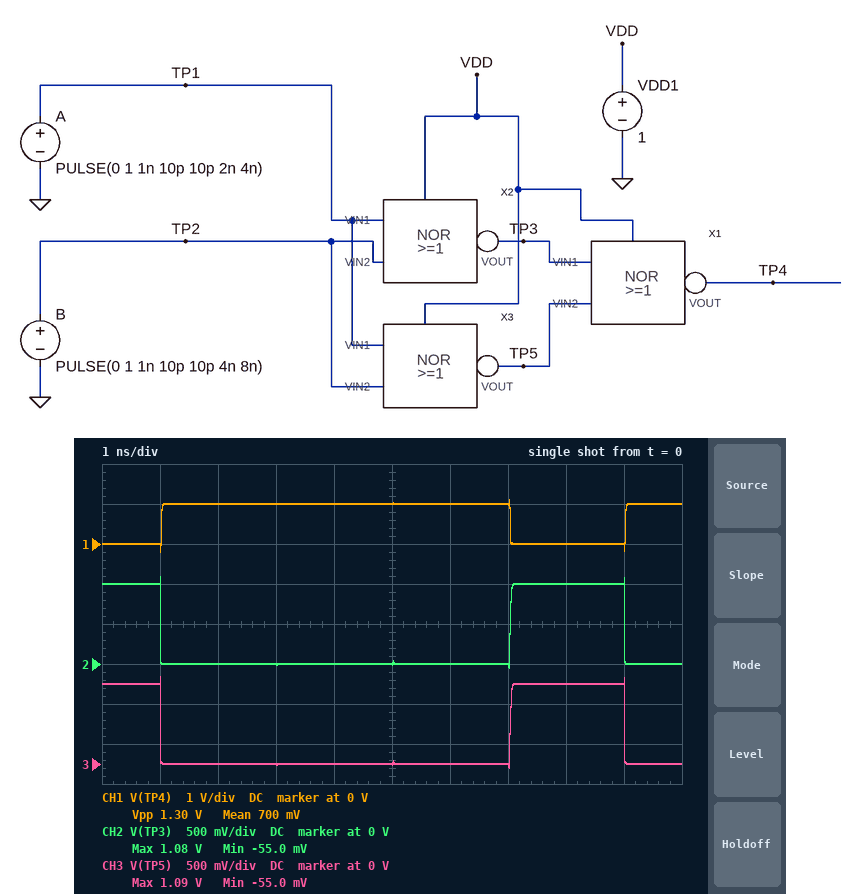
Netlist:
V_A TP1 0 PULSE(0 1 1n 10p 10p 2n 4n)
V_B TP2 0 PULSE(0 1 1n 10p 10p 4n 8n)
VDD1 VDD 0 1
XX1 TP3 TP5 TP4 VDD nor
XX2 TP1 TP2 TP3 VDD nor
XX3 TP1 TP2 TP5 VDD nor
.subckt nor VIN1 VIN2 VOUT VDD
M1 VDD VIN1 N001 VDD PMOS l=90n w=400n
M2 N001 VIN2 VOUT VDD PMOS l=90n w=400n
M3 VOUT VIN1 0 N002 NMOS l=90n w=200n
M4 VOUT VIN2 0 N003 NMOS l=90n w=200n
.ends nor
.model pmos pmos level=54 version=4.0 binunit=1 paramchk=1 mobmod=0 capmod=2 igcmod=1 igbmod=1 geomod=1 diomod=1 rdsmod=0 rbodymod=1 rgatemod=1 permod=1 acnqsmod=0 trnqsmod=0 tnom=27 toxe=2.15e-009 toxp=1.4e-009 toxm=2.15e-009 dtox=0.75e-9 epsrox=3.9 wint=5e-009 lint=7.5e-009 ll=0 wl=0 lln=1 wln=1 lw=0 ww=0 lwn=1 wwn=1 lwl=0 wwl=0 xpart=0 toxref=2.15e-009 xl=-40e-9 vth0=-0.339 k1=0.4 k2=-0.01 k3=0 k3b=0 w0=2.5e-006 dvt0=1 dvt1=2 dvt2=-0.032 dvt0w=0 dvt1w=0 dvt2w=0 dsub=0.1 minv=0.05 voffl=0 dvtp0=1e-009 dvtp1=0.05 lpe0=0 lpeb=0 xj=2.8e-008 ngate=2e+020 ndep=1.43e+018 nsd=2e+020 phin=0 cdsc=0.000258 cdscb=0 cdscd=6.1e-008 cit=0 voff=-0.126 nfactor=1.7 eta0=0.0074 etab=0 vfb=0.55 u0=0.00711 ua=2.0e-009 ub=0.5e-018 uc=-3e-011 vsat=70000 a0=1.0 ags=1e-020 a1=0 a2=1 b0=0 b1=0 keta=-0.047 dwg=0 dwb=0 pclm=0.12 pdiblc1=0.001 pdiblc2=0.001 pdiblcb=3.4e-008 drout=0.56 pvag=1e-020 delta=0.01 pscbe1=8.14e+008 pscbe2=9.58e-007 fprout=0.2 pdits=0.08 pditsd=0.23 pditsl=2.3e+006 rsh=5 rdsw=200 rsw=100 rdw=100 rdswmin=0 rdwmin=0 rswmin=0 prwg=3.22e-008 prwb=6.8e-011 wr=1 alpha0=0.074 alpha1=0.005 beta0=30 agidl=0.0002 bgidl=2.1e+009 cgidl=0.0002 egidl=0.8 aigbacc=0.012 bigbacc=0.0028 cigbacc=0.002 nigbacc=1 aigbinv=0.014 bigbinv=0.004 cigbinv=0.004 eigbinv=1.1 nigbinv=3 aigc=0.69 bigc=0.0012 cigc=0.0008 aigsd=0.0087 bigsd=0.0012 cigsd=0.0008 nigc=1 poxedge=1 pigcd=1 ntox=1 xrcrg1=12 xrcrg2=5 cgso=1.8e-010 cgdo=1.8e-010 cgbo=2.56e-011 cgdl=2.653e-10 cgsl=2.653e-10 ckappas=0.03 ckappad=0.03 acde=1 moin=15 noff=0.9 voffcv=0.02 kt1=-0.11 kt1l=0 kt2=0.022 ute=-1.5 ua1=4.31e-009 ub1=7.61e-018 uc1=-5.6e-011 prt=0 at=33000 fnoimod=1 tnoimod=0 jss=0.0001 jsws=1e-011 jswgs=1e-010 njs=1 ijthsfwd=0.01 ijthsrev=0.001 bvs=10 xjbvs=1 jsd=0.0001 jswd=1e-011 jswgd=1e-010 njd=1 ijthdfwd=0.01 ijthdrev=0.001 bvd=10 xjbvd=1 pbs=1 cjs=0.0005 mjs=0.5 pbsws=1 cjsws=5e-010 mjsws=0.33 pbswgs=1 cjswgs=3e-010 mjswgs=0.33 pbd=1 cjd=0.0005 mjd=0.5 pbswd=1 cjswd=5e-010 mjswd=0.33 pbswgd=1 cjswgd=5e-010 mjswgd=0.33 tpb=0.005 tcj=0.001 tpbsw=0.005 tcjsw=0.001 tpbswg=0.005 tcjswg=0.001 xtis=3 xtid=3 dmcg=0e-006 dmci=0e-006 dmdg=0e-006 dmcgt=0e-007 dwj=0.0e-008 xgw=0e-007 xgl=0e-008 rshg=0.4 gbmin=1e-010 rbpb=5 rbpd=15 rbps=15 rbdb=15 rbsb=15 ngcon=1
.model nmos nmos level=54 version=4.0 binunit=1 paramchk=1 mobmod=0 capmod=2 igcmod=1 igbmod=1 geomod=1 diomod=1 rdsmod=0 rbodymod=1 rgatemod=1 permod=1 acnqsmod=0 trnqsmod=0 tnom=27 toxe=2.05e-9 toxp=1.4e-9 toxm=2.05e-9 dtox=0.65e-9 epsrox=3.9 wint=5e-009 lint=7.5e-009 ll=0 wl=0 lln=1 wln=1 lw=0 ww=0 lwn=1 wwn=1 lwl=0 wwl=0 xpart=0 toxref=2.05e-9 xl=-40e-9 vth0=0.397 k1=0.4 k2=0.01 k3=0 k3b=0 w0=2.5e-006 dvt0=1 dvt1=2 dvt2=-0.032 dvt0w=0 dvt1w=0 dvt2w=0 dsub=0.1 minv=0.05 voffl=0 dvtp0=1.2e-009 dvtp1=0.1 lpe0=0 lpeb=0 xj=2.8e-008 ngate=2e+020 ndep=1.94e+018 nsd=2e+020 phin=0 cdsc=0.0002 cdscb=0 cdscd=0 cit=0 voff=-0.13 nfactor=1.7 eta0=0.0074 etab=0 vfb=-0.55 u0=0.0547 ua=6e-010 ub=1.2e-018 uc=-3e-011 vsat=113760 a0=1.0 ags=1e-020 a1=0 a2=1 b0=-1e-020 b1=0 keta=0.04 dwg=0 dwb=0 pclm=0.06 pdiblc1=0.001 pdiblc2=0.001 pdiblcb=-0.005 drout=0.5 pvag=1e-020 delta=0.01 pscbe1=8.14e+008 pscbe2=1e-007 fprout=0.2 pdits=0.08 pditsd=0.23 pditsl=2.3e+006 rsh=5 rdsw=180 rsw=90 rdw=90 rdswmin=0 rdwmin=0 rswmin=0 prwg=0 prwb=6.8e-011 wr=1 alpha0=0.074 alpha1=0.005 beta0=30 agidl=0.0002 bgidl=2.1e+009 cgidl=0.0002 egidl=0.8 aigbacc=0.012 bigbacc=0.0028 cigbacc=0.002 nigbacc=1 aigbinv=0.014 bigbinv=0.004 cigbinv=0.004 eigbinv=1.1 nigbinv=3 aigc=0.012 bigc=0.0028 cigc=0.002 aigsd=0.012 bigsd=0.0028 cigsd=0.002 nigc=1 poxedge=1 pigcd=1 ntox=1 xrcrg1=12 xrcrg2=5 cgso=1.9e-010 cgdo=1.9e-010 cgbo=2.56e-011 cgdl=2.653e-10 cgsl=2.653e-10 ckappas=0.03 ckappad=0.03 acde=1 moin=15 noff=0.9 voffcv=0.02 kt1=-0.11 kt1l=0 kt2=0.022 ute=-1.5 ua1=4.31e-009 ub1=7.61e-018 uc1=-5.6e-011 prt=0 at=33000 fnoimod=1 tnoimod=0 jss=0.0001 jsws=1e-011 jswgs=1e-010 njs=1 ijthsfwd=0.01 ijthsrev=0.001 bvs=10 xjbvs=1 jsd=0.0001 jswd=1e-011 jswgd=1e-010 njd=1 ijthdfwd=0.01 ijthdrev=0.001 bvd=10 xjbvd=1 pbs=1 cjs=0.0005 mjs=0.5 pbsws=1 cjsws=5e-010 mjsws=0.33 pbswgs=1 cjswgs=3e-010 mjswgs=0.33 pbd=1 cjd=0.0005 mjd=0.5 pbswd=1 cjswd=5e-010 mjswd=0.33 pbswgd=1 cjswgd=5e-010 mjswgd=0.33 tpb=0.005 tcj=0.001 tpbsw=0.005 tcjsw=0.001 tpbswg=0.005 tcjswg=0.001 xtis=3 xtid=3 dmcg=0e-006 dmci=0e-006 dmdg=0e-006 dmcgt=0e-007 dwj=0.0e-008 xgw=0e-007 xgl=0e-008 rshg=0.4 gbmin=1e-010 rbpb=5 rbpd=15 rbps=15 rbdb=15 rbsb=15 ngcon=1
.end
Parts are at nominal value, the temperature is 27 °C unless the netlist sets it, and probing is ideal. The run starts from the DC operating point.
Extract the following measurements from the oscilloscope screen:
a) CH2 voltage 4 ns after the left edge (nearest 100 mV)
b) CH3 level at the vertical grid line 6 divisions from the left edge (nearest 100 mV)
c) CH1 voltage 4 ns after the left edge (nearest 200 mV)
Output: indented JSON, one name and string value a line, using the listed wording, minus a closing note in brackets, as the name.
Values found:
{
  "CH2 voltage 4 ns after the left edge": "0 V",
  "CH3 level at the vertical grid line 6 divisions from the left edge": "0 V",
  "CH1 voltage 4 ns after the left edge": "1.0 V"
}
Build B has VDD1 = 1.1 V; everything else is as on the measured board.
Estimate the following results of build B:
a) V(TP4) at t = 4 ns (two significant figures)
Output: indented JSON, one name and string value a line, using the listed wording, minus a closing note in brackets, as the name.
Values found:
{
  "V(TP4) at t = 4 ns": "1.1 V"
}
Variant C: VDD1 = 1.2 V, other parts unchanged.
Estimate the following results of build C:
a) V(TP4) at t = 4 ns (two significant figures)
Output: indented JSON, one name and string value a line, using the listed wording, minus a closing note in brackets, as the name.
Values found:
{
  "V(TP4) at t = 4 ns": "1.2 V"
}
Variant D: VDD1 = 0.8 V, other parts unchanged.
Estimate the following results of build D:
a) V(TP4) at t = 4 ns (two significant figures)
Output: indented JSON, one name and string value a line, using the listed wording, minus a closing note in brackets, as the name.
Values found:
{
  "V(TP4) at t = 4 ns": "800 mV"
}
